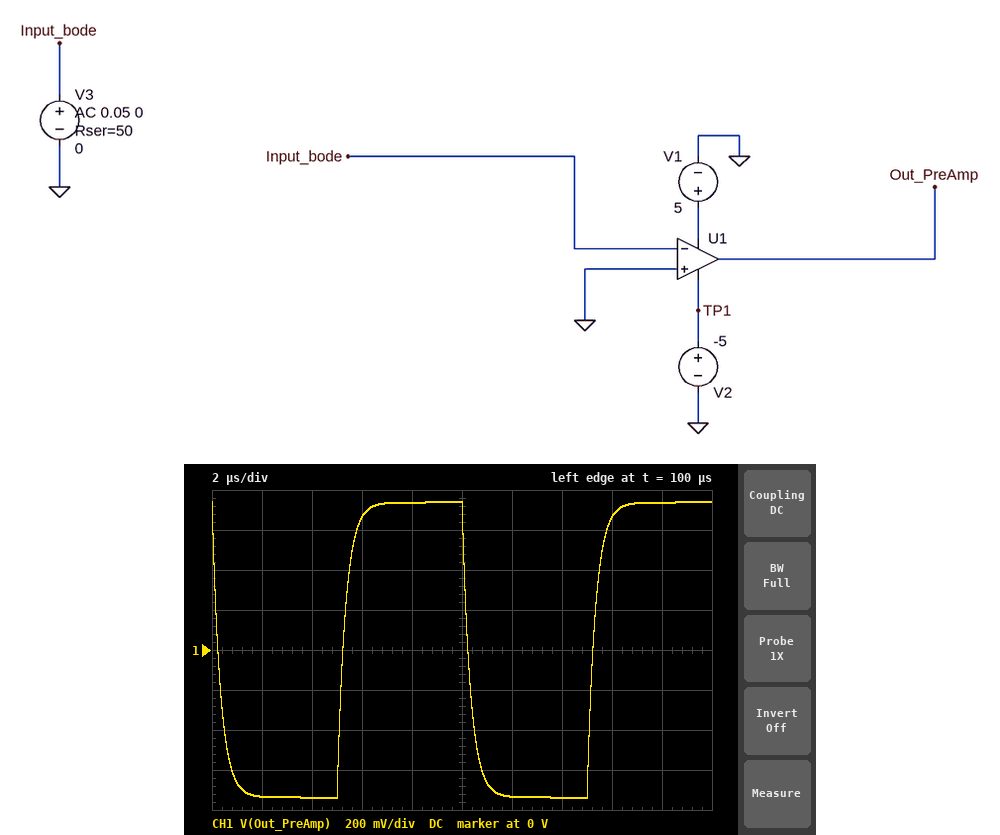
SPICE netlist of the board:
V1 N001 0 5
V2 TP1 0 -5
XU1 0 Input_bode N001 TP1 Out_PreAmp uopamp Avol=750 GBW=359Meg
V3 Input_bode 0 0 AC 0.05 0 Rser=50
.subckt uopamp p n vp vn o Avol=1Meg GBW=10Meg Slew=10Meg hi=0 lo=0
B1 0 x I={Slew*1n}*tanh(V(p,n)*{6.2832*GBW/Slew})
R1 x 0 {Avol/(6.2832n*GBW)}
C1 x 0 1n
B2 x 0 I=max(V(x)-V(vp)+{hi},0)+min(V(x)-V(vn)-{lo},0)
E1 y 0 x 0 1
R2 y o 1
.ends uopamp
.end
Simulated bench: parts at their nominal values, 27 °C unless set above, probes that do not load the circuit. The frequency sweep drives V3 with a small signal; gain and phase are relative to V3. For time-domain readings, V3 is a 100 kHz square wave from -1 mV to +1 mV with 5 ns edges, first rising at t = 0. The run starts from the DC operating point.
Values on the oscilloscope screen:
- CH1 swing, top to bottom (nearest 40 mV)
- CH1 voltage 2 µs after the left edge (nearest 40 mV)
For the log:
1.48 V
-720 mV
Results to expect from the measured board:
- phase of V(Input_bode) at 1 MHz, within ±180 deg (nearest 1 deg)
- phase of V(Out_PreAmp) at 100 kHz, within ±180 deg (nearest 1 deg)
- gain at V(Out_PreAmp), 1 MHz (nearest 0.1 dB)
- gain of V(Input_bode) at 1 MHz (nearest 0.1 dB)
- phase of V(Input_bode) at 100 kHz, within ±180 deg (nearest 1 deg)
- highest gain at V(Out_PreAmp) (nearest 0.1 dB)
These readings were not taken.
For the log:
0 deg
168 deg
50.2 dB
0 dB
0 deg
57.5 dB
